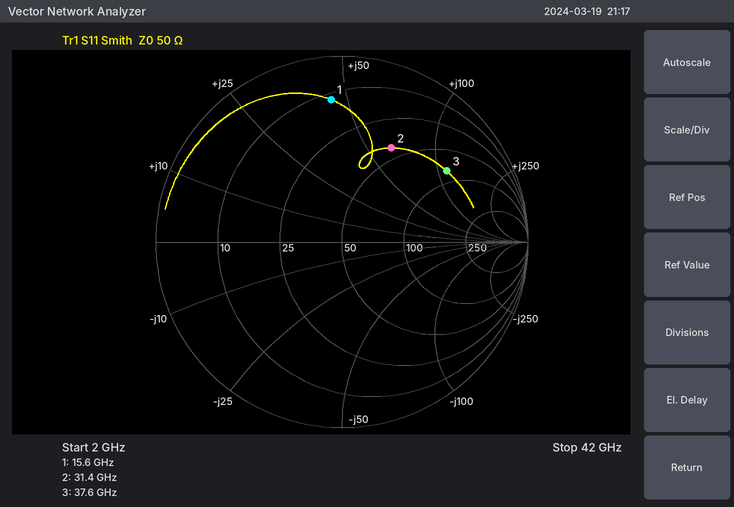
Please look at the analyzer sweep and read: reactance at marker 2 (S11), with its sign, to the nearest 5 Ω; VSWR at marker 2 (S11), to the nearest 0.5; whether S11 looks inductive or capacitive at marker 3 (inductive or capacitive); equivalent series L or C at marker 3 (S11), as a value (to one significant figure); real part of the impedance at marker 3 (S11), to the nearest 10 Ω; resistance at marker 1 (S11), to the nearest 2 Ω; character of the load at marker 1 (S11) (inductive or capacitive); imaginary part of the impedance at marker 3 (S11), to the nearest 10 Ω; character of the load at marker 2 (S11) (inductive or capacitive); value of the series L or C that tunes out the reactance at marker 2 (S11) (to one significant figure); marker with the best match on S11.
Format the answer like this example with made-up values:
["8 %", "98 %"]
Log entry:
["+65 Ω", "3.5", "inductive", "500 pH", "80 Ω", "12 Ω", "inductive", "+110 Ω", "inductive", "80 fF", "marker 2"]
